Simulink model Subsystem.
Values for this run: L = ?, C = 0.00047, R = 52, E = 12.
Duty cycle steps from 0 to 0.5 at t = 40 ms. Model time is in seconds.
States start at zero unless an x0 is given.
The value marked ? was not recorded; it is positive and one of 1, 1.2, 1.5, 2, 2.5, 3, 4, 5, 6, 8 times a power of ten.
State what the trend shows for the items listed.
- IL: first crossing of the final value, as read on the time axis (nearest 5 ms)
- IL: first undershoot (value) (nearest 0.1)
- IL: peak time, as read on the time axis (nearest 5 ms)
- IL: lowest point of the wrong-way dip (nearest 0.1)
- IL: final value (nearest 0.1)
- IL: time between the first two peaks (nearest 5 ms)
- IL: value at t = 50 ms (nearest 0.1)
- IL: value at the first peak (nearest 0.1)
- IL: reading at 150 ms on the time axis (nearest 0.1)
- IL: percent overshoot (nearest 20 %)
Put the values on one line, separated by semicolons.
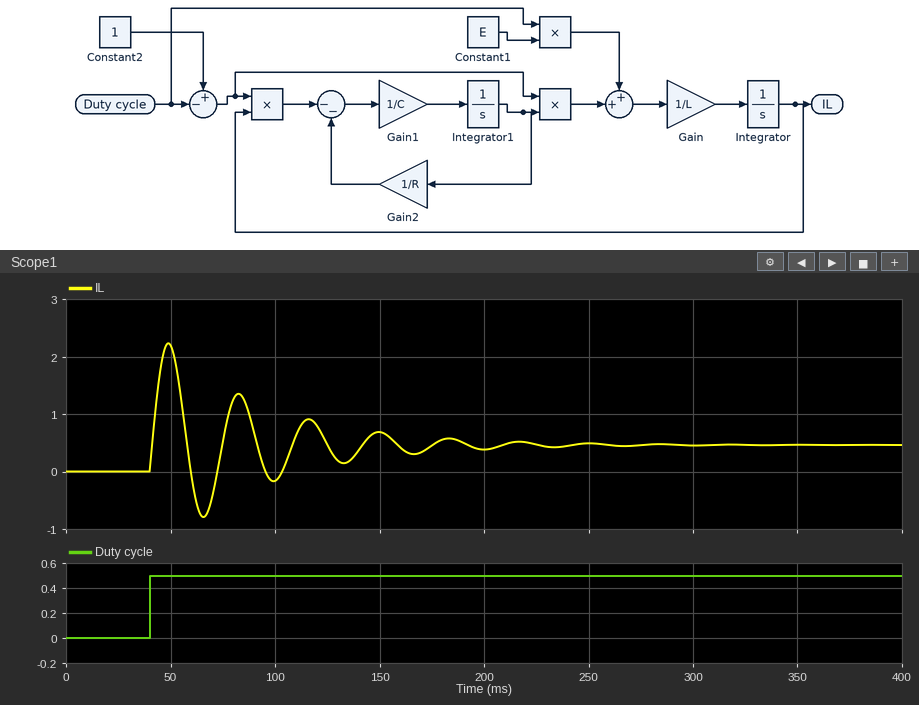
40 ms; -0.8; 50 ms; -0.8; 0.5; 35 ms; 2.2; 2.2; 0.7; 380 %
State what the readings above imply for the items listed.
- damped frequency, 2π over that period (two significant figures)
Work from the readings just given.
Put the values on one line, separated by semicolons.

0.18 rad/ms
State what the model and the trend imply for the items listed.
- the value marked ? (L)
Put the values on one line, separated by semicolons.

0.015
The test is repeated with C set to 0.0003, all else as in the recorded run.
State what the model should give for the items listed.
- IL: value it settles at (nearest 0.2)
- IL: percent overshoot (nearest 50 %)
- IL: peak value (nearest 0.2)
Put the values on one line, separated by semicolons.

0.4; 300 %; 1.8
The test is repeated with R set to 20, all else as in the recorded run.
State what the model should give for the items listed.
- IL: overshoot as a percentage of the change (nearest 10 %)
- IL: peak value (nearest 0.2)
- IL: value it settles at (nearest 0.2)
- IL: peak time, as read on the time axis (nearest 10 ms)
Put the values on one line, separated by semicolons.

100 %; 2.4; 1.2; 50 ms
